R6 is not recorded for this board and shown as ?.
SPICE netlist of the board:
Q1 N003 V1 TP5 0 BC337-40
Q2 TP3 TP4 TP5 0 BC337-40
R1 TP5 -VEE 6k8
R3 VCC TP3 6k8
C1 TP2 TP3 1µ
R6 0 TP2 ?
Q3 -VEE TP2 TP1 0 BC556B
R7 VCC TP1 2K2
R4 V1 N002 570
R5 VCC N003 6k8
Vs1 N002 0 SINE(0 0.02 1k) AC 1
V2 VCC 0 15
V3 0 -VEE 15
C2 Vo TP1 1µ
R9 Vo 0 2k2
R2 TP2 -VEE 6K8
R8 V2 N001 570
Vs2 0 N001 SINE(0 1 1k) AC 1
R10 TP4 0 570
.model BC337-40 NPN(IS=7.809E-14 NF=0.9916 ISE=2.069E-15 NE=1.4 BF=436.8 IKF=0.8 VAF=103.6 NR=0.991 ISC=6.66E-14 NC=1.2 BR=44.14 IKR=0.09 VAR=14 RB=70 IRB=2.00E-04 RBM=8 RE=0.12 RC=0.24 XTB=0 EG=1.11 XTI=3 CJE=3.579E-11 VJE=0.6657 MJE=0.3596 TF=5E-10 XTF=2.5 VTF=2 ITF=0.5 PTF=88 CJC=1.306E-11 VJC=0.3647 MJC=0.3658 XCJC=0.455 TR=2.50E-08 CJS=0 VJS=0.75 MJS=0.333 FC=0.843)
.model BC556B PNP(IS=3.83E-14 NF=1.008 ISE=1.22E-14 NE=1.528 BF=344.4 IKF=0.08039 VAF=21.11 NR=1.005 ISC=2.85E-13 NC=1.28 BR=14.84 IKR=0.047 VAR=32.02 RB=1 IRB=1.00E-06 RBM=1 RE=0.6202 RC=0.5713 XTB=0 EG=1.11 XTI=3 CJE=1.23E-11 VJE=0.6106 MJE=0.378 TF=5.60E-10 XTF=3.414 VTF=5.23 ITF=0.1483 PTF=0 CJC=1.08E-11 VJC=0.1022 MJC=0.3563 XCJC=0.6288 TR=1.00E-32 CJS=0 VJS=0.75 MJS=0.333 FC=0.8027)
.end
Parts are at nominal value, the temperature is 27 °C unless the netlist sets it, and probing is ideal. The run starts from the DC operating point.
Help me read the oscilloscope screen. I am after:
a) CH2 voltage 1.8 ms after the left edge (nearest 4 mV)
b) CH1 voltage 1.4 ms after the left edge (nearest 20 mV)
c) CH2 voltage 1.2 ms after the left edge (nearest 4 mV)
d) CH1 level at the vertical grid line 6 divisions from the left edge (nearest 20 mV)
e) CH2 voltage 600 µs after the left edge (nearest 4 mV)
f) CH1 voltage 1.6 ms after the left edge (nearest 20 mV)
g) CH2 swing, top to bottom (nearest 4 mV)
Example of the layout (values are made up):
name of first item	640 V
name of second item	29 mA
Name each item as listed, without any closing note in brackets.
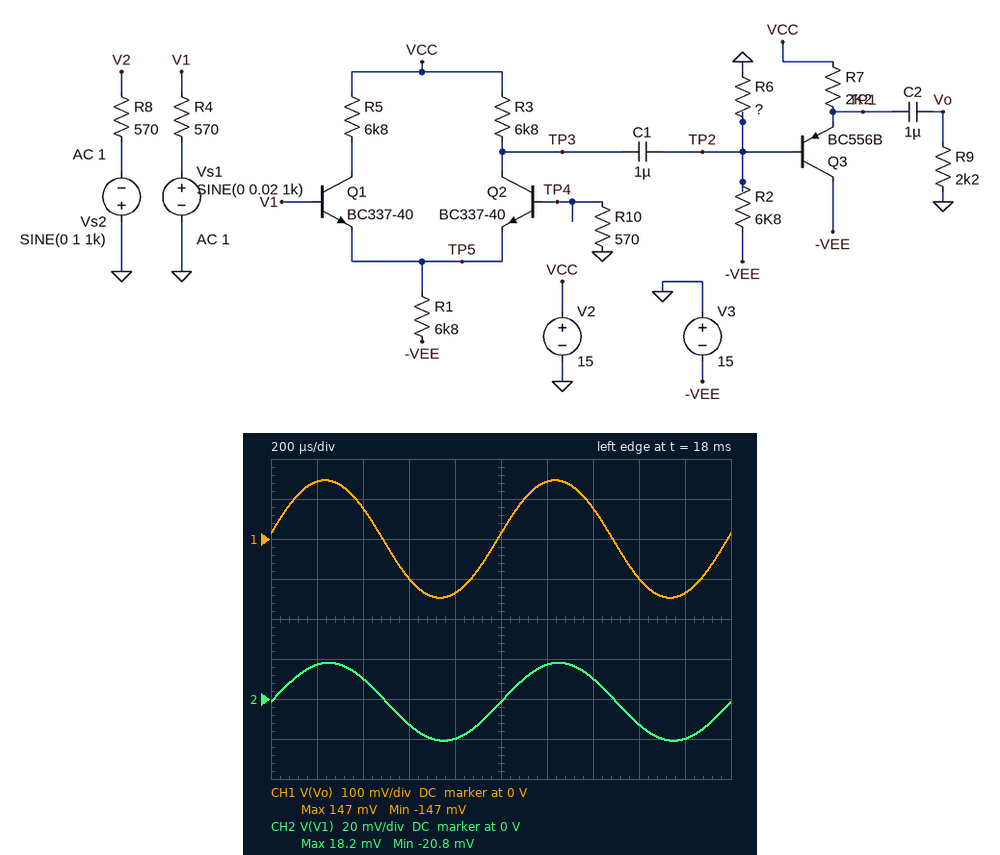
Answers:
CH2 voltage 1.8 ms after the left edge	-20 mV
CH1 voltage 1.4 ms after the left edge	80 mV
CH2 voltage 1.2 ms after the left edge	16 mV
CH1 level at the vertical grid line 6 divisions from the left edge	140 mV
CH2 voltage 600 µs after the left edge	-12 mV
CH1 voltage 1.6 ms after the left edge	-100 mV
CH2 swing, top to bottom	40 mV
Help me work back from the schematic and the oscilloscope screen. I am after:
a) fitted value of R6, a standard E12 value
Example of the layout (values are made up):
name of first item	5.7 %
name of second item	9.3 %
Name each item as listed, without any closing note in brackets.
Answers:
fitted value of R6, a standard E12 value	470 Ω
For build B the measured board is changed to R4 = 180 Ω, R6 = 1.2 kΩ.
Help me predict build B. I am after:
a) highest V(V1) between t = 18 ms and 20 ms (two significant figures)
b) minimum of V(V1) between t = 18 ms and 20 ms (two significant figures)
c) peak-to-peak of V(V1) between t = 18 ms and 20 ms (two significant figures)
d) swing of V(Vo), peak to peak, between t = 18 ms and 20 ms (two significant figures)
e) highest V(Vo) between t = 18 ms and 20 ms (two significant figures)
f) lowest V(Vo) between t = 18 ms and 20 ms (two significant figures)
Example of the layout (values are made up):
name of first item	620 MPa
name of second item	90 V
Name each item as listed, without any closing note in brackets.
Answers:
highest V(V1) between t = 18 ms and 20 ms	19 mV
minimum of V(V1) between t = 18 ms and 20 ms	-20 mV
peak-to-peak of V(V1) between t = 18 ms and 20 ms	40 mV
swing of V(Vo), peak to peak, between t = 18 ms and 20 ms	640 mV
highest V(Vo) between t = 18 ms and 20 ms	320 mV
lowest V(Vo) between t = 18 ms and 20 ms	-320 mV
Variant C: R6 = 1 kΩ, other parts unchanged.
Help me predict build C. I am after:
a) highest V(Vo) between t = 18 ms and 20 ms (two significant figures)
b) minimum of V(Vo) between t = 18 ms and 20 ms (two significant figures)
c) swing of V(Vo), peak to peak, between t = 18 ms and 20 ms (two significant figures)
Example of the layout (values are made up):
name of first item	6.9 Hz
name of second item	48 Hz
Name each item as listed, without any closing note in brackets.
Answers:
highest V(Vo) between t = 18 ms and 20 ms	270 mV
minimum of V(Vo) between t = 18 ms and 20 ms	-270 mV
swing of V(Vo), peak to peak, between t = 18 ms and 20 ms	550 mV
